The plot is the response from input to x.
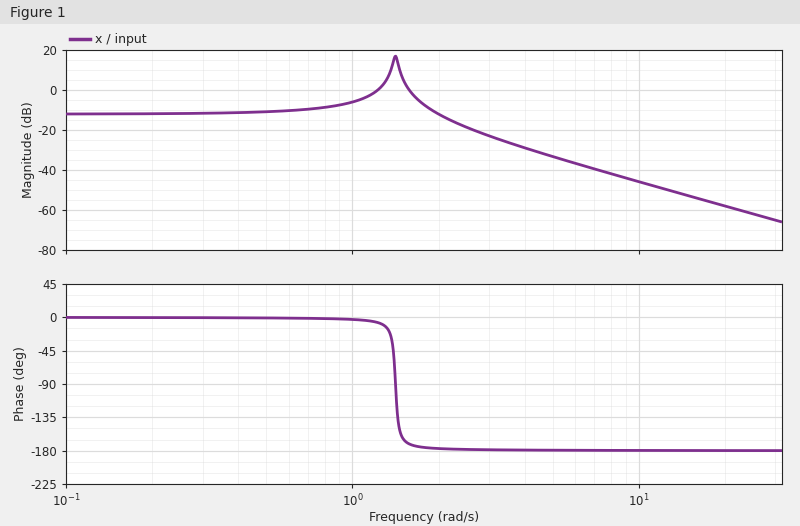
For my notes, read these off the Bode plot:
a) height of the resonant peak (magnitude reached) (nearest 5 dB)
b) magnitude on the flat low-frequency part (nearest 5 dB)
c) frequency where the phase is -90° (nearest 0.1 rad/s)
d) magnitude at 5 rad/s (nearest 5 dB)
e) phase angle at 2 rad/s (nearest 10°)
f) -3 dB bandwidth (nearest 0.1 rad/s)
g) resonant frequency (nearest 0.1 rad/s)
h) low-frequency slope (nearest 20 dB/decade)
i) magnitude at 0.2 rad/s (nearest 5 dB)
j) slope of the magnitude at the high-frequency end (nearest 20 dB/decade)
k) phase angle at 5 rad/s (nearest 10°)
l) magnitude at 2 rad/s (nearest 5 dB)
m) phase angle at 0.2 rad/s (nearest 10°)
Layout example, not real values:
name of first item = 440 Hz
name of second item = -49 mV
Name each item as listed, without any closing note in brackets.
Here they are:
height of the resonant peak (magnitude reached) = 15 dB
magnitude on the flat low-frequency part = -10 dB
frequency where the phase is -90° = 1.4 rad/s
magnitude at 5 rad/s = -35 dB
phase angle at 2 rad/s = -180°
-3 dB bandwidth = 2.2 rad/s
resonant frequency = 1.4 rad/s
low-frequency slope = 0 dB/decade
magnitude at 0.2 rad/s = -10 dB
slope of the magnitude at the high-frequency end = -40 dB/decade
phase angle at 5 rad/s = -180°
magnitude at 2 rad/s = -10 dB
phase angle at 0.2 rad/s = 0°
